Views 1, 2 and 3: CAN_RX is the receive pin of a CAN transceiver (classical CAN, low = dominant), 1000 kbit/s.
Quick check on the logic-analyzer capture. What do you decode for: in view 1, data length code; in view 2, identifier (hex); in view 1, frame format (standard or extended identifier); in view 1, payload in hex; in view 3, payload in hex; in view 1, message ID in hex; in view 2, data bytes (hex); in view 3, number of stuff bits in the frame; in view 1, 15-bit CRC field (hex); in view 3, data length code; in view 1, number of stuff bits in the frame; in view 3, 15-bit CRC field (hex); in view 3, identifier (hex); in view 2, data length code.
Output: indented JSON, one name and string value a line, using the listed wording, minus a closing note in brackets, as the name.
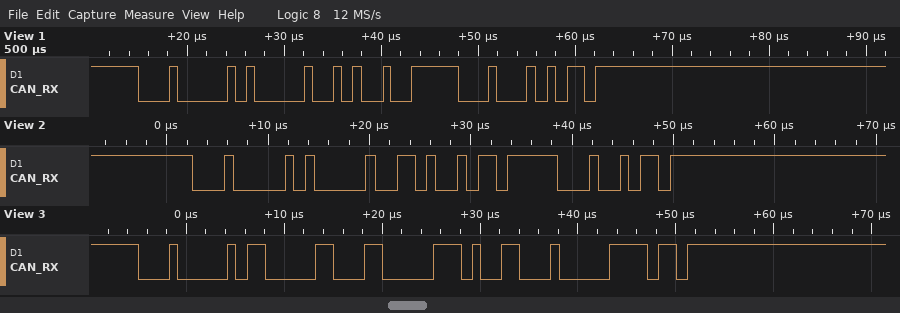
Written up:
{
  "in view 1, data length code": "1",
  "in view 2, identifier": "0x102",
  "in view 1, frame format": "standard",
  "in view 1, payload in hex": "49",
  "in view 3, payload in hex": "30 69",
  "in view 1, message ID in hex": "0x102",
  "in view 2, data bytes": "A5",
  "in view 3, number of stuff bits in the frame": "4",
  "in view 1, 15-bit CRC field": "0x7915",
  "in view 3, data length code": "2",
  "in view 1, number of stuff bits in the frame": "3",
  "in view 3, 15-bit CRC field": "0x441D",
  "in view 3, identifier": "0x103",
  "in view 2, data length code": "1"
}
